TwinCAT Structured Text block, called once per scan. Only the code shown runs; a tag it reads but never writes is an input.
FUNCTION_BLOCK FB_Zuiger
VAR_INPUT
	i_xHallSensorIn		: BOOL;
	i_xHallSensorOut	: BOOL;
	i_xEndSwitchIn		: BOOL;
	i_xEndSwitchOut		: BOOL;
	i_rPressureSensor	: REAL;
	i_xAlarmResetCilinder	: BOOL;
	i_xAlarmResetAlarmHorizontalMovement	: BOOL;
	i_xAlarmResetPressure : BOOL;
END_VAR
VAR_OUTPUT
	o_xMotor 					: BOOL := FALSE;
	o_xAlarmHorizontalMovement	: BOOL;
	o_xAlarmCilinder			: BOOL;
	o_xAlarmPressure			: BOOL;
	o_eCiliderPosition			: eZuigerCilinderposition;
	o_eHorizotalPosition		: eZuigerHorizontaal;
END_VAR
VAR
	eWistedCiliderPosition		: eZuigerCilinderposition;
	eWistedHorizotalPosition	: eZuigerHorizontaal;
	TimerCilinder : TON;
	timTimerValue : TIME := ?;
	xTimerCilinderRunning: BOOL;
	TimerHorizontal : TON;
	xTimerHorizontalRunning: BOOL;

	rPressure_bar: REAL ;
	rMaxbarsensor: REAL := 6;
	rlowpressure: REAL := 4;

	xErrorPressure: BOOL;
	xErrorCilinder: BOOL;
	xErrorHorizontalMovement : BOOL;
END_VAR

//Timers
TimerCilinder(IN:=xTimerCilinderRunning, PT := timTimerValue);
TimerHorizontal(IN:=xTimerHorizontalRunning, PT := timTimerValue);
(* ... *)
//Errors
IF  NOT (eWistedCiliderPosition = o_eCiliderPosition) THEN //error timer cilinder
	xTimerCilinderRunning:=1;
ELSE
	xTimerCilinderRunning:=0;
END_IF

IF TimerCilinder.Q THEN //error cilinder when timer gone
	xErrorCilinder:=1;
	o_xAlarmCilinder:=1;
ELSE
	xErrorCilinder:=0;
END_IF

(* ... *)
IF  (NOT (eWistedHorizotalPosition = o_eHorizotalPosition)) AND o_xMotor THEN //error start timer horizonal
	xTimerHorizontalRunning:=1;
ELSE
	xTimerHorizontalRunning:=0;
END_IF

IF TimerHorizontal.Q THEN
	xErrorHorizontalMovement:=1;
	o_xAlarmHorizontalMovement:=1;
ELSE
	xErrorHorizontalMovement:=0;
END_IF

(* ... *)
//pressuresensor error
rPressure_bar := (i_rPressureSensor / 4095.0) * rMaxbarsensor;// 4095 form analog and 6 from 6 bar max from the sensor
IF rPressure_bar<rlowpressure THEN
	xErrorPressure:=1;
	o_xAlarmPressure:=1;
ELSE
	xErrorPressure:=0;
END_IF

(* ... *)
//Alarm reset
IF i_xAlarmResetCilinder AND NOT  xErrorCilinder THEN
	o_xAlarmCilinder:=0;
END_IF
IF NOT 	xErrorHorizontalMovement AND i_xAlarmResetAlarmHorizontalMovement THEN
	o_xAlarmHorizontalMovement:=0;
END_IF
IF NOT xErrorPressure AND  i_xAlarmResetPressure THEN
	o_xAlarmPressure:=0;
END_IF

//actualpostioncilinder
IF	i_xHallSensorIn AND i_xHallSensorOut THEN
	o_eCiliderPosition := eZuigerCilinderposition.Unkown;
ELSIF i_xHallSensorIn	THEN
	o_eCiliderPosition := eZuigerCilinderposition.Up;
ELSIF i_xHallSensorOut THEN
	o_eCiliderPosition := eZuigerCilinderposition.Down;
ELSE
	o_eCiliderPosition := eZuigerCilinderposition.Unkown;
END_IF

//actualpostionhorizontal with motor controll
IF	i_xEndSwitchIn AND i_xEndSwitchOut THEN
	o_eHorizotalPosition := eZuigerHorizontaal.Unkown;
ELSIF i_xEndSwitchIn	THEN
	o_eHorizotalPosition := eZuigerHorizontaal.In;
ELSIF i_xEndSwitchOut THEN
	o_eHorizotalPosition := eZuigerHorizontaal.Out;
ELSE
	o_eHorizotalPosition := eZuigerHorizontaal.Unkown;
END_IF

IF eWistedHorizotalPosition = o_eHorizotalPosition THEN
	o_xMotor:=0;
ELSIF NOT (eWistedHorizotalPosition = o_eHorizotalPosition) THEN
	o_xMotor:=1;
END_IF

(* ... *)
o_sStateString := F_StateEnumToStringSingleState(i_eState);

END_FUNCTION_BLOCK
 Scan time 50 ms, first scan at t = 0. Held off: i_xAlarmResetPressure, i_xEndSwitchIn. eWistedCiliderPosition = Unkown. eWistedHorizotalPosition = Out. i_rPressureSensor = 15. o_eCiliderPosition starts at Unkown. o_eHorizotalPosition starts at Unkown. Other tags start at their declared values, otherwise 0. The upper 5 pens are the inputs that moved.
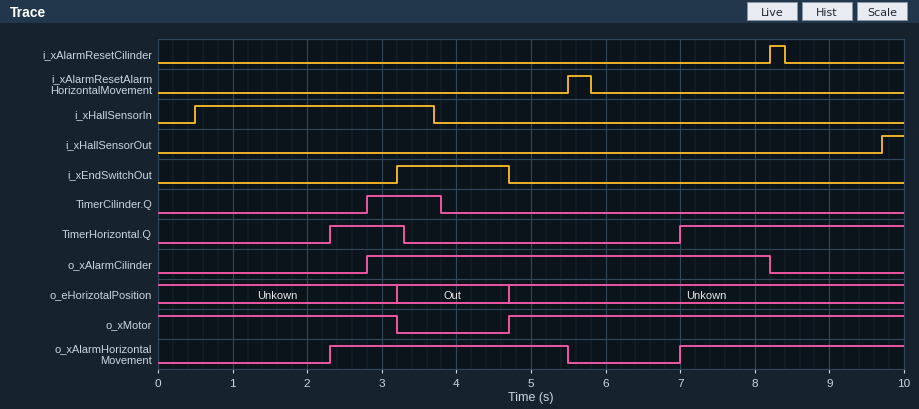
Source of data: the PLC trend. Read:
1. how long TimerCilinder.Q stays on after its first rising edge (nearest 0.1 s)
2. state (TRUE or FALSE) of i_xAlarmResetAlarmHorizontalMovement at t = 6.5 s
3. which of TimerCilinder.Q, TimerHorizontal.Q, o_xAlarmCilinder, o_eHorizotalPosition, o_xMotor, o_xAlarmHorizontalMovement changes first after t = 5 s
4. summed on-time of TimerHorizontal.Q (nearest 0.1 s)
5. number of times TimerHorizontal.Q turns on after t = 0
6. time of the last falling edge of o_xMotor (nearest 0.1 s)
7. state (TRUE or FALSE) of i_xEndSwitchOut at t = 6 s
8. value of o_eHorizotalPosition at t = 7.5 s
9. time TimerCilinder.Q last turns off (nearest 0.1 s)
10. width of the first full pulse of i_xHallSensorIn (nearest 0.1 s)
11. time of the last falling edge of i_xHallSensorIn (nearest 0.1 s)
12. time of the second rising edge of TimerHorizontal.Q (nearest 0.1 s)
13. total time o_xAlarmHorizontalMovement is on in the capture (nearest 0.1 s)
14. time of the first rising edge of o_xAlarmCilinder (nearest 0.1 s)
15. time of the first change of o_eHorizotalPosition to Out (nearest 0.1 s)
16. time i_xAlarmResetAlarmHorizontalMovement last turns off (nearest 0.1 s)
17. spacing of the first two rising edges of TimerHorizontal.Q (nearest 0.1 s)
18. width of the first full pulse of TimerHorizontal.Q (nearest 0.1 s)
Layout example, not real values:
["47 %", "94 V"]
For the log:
["1.0 s", "FALSE", "o_xAlarmHorizontalMovement", "4.0 s", "2", "3.2 s", "FALSE", "Unkown", "3.8 s", "3.2 s", "3.7 s", "7.0 s", "6.2 s", "2.8 s", "3.2 s", "5.8 s", "4.7 s", "1.0 s"]
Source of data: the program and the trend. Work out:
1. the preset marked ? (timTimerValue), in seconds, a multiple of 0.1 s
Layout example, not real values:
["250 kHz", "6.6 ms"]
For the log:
["2.2 s"]
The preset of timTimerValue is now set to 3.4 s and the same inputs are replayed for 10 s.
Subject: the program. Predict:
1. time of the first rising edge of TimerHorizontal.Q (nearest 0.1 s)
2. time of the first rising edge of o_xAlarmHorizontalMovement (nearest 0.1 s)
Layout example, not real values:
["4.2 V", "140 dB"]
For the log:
["8.2 s", "8.2 s"]
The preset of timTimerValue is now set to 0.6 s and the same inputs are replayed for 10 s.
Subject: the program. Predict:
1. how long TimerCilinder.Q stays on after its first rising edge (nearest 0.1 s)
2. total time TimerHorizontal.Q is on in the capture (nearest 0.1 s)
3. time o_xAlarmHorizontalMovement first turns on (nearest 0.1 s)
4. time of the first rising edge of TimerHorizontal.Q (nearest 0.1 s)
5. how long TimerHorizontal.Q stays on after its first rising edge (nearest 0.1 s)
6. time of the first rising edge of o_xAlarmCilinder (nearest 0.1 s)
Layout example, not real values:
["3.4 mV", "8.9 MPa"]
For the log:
["2.6 s", "7.2 s", "0.7 s", "0.7 s", "2.6 s", "1.2 s"]
